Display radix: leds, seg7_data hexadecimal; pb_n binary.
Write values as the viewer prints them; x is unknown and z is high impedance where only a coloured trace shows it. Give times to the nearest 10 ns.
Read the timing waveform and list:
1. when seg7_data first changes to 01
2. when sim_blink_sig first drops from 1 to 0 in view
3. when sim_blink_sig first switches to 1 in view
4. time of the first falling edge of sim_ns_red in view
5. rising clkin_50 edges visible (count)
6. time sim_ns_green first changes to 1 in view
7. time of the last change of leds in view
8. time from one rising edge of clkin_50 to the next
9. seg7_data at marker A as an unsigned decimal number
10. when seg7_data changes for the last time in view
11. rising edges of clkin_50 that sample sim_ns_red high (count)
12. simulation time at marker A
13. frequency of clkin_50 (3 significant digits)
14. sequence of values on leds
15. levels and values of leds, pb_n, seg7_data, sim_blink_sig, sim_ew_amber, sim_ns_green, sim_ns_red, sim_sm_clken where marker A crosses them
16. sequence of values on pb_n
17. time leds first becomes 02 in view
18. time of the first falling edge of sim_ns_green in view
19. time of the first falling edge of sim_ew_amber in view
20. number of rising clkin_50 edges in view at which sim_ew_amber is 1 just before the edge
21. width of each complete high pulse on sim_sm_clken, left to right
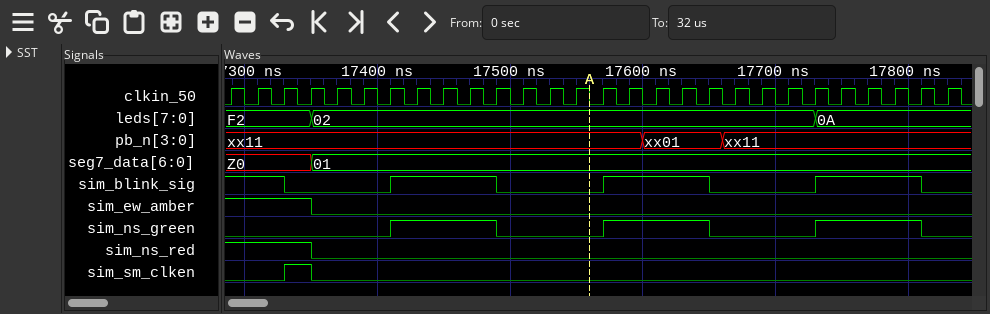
17350 ns
17330 ns
17410 ns
17350 ns
28
17410 ns
17730 ns
20 ns
1
17350 ns
4
17560 ns
50.0 MHz
F2, 02, 0A
leds=02, pb_n=xx11, seg7_data=01, sim_blink_sig=0, sim_ew_amber=0, sim_ns_green=0, sim_ns_red=0, sim_sm_clken=0
xx11, xx01, xx11
17350 ns
17490 ns
17350 ns
4
20 ns
